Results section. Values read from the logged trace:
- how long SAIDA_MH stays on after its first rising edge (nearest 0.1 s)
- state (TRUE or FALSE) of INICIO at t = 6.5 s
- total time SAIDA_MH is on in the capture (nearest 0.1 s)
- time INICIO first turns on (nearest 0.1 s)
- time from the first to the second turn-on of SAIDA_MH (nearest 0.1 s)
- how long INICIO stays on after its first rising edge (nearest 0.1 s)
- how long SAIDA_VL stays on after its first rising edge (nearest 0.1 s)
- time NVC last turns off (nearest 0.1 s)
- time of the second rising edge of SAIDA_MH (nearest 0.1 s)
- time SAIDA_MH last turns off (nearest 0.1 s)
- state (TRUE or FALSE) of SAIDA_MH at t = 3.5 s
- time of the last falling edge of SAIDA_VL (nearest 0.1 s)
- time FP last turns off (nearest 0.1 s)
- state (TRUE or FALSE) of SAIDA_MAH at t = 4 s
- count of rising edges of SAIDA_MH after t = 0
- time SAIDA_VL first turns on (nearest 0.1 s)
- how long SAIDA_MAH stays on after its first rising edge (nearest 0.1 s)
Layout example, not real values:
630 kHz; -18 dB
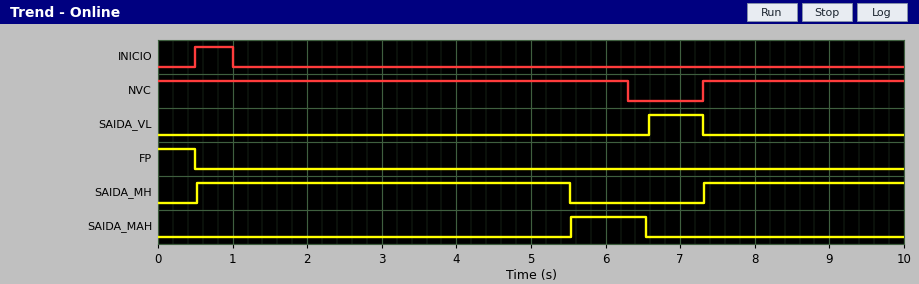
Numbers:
5.0 s; FALSE; 7.7 s; 0.5 s; 6.8 s; 0.5 s; 0.7 s; 6.3 s; 7.3 s; 5.5 s; TRUE; 7.3 s; 0.5 s; FALSE; 2; 6.6 s; 1.0 s
